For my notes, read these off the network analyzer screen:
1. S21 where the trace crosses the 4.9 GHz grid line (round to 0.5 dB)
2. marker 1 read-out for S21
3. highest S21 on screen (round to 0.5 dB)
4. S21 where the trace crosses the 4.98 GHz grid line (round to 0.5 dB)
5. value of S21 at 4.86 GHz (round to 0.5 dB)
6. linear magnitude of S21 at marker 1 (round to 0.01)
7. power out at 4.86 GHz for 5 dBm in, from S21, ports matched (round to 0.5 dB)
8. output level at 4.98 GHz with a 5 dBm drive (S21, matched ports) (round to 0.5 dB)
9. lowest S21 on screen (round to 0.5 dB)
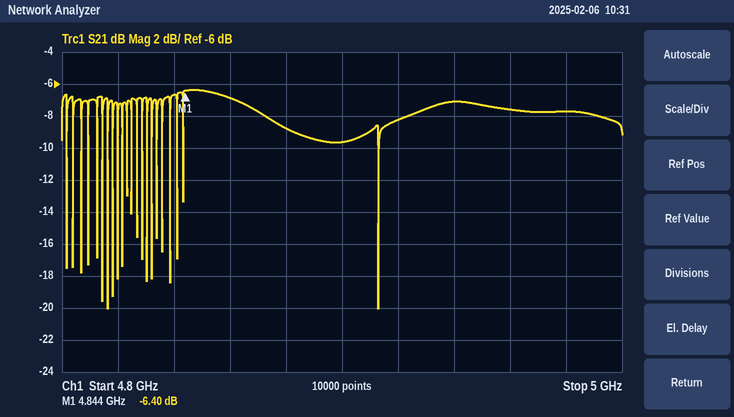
-9.5 dB
-6.40 dB
-6.5 dB
-7.5 dB
-7.0 dB
0.48
-2.0 dBm
-2.5 dBm
-20.0 dB
